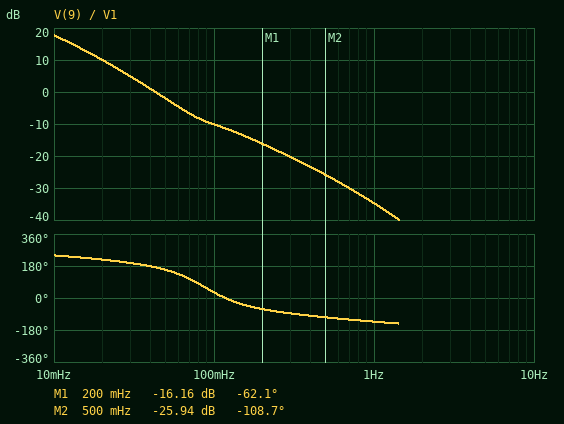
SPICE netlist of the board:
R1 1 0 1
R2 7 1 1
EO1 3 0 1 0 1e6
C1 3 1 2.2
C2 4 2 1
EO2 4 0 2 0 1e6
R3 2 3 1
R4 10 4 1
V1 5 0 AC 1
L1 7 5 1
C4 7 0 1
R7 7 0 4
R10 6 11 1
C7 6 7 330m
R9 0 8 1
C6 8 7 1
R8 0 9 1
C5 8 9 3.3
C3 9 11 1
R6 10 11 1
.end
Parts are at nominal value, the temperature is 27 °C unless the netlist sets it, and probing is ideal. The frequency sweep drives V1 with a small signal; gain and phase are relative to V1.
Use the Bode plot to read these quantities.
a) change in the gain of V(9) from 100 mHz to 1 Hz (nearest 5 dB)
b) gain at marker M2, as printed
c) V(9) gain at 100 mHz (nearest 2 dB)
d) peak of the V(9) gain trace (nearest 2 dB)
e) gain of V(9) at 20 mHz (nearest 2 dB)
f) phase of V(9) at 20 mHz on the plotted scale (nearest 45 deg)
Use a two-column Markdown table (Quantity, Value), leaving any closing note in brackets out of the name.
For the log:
| Quantity | Value |
|---|---|
| change in the gain of V(9) from 100 mHz to 1 Hz | -25 dB |
| gain at marker M2, as printed | -25.94 dB |
| V(9) gain at 100 mHz | -10 dB |
| peak of the V(9) gain trace | 18 dB |
| gain of V(9) at 20 mHz | 10 dB |
| phase of V(9) at 20 mHz on the plotted scale | 225 deg |
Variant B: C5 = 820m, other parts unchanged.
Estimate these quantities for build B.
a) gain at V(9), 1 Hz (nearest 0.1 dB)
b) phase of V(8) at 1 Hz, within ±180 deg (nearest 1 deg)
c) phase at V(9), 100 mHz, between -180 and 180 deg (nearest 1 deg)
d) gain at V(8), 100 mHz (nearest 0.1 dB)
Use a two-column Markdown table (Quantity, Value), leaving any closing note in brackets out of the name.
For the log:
| Quantity | Value |
|---|---|
| gain at V(9), 1 Hz | -35.5 dB |
| phase of V(8) at 1 Hz, within ±180 deg | -140 deg |
| phase at V(9), 100 mHz, between -180 and 180 deg | 62 deg |
| gain at V(8), 100 mHz | -9.7 dB |
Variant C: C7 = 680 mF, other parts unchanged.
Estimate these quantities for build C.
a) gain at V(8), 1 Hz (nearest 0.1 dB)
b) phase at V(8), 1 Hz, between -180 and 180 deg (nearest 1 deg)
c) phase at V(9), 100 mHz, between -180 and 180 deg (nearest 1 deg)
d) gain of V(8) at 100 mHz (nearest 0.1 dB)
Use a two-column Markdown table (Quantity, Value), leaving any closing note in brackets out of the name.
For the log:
| Quantity | Value |
|---|---|
| gain at V(8), 1 Hz | -34.7 dB |
| phase at V(8), 1 Hz, between -180 and 180 deg | -137 deg |
| phase at V(9), 100 mHz, between -180 and 180 deg | 16 deg |
| gain of V(8) at 100 mHz | -12.1 dB |
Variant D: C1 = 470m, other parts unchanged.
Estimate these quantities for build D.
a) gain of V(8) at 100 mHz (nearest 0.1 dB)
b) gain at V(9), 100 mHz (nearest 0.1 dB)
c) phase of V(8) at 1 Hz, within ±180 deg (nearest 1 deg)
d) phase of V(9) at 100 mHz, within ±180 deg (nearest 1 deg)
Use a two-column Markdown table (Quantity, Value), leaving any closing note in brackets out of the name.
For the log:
| Quantity | Value |
|---|---|
| gain of V(8) at 100 mHz | -9.2 dB |
| gain at V(9), 100 mHz | -2.8 dB |
| phase of V(8) at 1 Hz, within ±180 deg | -136 deg |
| phase of V(9) at 100 mHz, within ±180 deg | 62 deg |
